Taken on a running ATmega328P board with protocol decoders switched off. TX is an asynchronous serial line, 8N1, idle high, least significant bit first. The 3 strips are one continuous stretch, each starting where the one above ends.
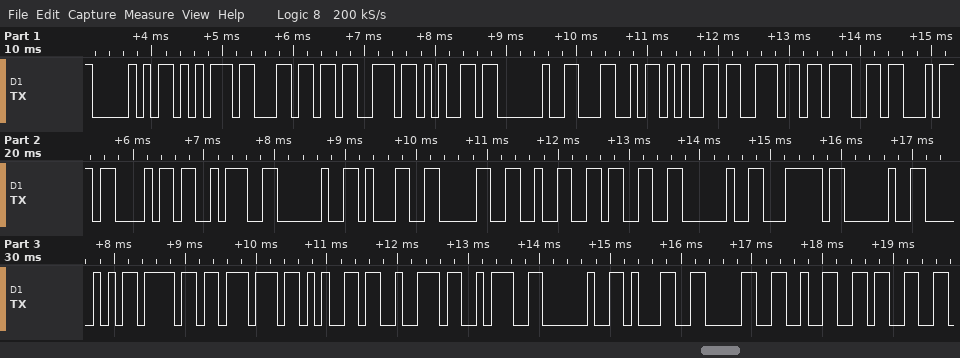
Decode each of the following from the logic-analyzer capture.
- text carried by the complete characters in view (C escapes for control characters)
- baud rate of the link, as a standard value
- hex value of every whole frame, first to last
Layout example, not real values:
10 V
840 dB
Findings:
"Pulse Length: 1023 | Power: 1023"
9600 baud
50 75 6C 73 65 20 4C 65 6E 67 74 68 3A 20 31 30 32 33 20 7C 20 50 6F 77 65 72 3A 20 31 30 32 33
